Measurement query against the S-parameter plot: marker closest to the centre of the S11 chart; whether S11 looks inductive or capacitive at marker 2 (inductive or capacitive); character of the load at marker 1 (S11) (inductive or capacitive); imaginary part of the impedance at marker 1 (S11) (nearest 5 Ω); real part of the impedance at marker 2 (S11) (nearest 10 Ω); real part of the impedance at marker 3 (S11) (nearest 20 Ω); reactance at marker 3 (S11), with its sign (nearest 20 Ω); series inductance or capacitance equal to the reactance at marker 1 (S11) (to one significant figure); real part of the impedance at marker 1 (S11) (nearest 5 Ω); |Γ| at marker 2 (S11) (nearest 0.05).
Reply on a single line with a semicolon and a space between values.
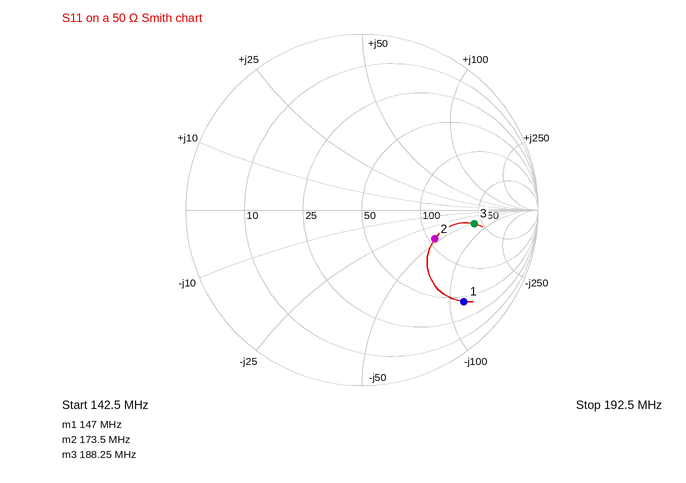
marker 2; capacitive; capacitive; -115 Ω; 110 Ω; 220 Ω; -60 Ω; 9 pF; 45 Ω; 0.45
